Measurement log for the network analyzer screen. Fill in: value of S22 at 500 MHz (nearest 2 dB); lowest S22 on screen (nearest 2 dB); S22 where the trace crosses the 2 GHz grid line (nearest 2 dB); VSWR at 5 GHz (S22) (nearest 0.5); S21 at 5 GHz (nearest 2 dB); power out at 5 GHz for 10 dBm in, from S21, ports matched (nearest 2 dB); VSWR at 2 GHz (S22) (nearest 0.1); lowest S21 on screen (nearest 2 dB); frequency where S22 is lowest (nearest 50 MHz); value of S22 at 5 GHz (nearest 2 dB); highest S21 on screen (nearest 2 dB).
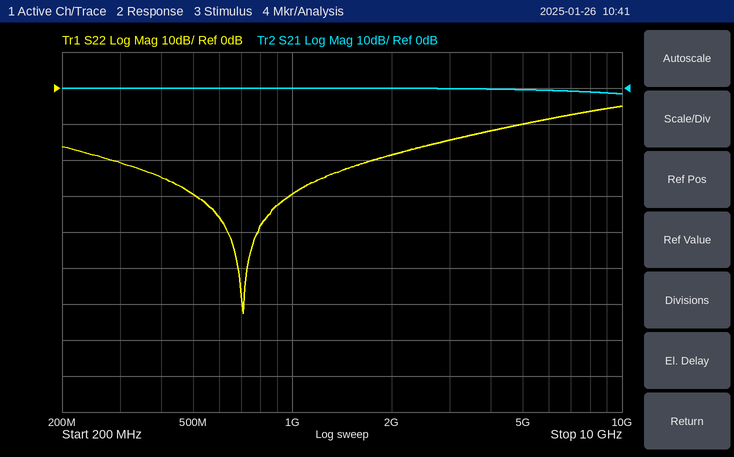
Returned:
-30 dB
-62 dB
-18 dB
2.0
0 dB
10 dBm
1.3
-2 dB
700 MHz
-10 dB
0 dB
